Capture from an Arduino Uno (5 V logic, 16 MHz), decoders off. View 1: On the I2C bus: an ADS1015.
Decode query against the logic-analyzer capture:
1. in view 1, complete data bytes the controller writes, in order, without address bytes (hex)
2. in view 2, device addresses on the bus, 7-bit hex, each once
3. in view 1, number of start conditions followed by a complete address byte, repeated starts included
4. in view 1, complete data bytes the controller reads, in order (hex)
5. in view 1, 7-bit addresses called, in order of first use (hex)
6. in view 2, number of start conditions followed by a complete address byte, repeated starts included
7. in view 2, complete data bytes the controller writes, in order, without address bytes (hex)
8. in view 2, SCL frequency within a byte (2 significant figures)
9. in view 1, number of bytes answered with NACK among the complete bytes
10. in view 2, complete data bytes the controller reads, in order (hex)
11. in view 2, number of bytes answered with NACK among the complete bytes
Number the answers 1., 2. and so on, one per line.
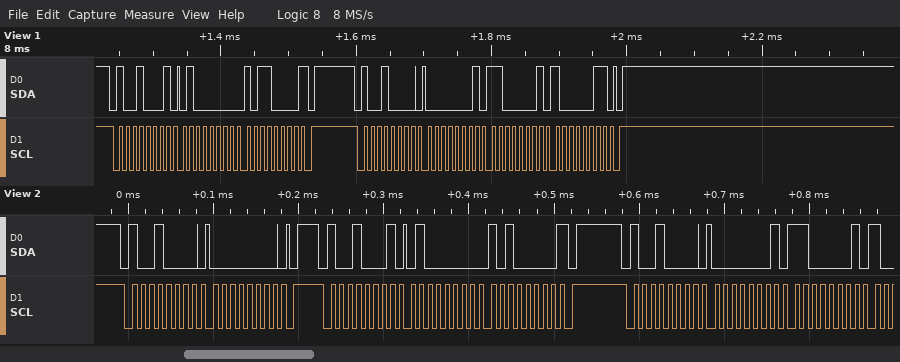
1. 01 C1 83
2. 0x48
3. 2
4. 40 B0
5. 0x48
6. 3
7. 00 01 C1
8. 100 kHz
9. 1
10. 40 A0
11. 1
